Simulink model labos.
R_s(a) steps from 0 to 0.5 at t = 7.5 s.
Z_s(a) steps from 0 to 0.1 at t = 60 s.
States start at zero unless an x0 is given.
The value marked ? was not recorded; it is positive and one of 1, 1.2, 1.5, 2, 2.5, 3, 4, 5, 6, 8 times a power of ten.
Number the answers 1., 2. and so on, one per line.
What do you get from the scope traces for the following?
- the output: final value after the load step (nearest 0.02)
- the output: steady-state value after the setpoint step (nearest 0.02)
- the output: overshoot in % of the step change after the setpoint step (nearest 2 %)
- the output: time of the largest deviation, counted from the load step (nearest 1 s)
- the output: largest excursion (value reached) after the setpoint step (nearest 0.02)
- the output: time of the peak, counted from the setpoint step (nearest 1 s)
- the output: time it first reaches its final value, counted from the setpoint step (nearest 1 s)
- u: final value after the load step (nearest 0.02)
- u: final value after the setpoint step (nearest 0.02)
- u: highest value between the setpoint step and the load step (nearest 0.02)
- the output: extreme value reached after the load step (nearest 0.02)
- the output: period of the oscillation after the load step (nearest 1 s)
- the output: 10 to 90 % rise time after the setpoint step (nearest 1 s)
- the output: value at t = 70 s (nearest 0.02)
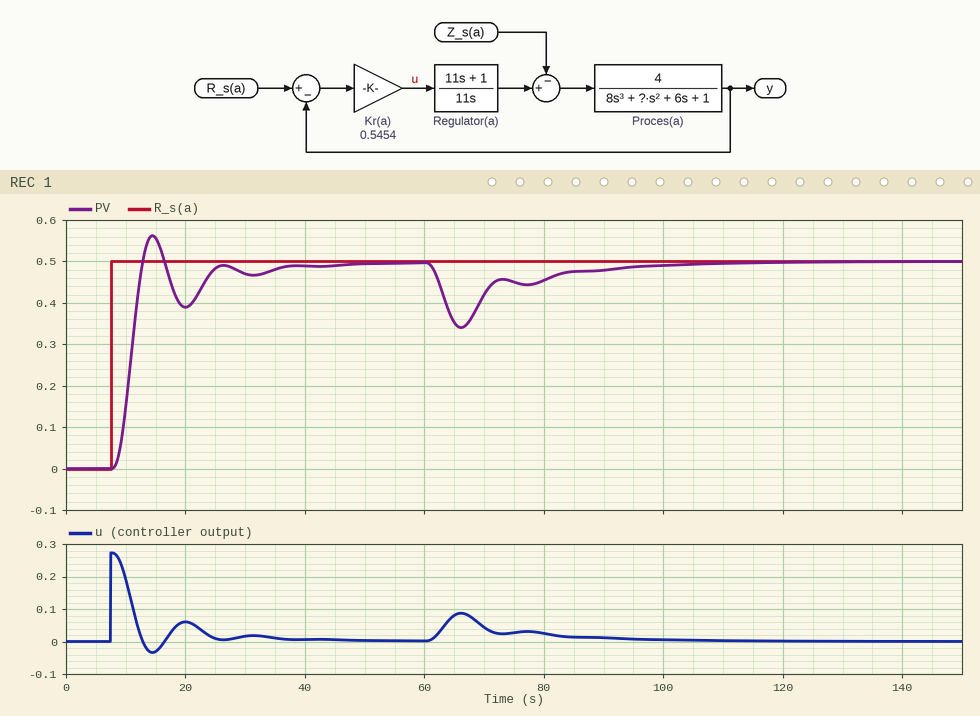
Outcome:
1. 0.50
2. 0.50
3. 12 %
4. 6 s
5. 0.56
6. 7 s
7. 5 s
8. 0.00
9. 0.00
10. 0.28
11. 0.34
12. 11 s
13. 3 s
14. 0.42
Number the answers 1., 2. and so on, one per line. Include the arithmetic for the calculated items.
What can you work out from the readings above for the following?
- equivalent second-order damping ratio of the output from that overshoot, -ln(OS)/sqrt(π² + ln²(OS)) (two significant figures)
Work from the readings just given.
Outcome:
1. ln(0.12) = -2.120; 2.120 / sqrt(9.870 + 4.496) = 0.56
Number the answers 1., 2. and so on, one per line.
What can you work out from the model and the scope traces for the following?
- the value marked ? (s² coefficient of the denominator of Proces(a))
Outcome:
1. 12
